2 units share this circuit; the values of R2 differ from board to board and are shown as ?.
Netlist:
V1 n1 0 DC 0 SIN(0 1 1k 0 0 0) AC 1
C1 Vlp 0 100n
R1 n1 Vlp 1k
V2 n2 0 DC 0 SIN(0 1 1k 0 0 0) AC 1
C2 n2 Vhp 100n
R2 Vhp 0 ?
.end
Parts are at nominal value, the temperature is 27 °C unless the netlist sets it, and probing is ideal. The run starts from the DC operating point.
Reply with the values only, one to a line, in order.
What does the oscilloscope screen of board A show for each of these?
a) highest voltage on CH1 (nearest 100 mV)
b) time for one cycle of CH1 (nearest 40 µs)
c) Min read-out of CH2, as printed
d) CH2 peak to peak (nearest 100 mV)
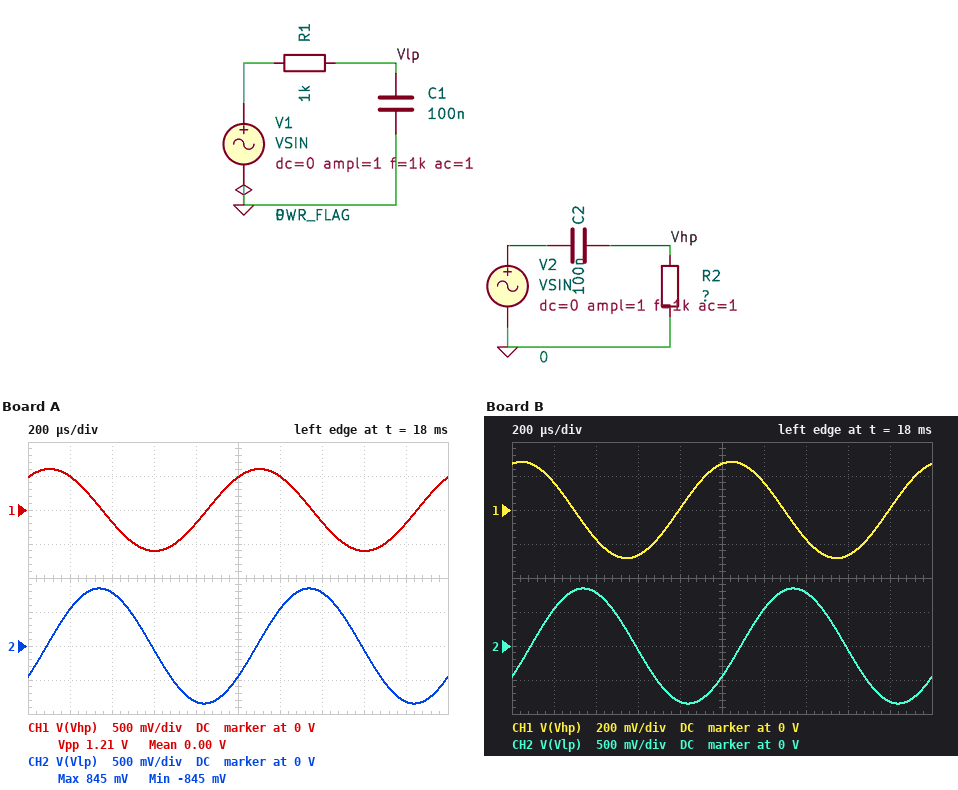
600 mV
1.00 ms
-845 mV
1.7 V
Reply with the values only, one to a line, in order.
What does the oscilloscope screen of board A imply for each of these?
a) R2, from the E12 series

1.2 kΩ
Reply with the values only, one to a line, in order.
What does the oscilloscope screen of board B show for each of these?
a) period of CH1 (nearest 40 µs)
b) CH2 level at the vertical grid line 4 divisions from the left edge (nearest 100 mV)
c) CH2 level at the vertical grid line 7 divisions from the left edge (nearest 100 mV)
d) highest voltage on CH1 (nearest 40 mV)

1.00 ms
-800 mV
800 mV
280 mV
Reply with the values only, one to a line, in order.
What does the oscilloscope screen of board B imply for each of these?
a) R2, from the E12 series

470 Ω
